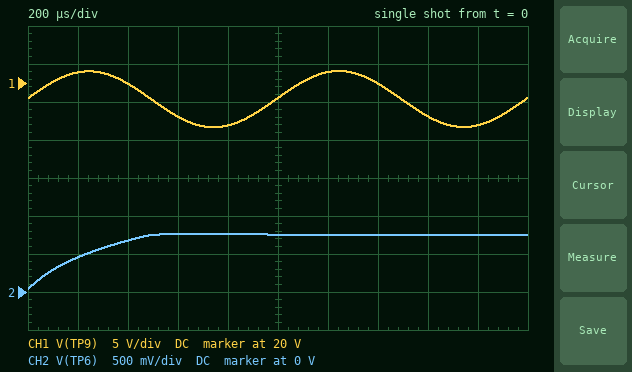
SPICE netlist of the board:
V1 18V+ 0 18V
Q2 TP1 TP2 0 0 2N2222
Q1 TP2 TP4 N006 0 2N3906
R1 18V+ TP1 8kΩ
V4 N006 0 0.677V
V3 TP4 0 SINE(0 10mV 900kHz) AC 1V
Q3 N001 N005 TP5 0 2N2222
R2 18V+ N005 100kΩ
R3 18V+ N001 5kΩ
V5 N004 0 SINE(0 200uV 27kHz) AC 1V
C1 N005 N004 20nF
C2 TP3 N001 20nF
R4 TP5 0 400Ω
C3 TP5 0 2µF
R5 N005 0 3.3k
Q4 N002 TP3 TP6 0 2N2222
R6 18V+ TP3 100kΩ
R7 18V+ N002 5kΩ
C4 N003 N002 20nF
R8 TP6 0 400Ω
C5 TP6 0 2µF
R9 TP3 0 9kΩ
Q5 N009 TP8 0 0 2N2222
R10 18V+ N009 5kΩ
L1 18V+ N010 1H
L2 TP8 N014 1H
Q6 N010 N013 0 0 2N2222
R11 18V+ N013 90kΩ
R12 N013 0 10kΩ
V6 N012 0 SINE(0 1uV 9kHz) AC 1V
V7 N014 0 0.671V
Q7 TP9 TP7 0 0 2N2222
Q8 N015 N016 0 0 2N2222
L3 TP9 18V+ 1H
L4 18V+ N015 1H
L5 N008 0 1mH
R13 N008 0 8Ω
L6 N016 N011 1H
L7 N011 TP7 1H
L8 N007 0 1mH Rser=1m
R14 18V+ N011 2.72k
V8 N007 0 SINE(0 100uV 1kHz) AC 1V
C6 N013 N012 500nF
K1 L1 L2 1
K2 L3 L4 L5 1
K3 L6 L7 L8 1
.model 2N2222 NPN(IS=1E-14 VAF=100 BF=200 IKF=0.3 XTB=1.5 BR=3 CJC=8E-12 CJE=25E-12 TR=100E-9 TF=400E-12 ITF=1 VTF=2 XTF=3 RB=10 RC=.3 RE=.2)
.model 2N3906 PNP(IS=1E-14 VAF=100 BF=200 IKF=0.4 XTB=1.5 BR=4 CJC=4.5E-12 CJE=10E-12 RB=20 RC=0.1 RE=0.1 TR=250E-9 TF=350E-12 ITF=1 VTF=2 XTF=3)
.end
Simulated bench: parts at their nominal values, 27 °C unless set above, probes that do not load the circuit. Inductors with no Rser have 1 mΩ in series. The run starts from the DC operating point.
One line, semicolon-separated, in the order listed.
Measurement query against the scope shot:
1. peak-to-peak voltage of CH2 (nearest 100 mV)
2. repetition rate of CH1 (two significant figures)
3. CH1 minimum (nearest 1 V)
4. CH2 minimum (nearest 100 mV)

700 mV; 1.0 kHz; 14 V; 0 V
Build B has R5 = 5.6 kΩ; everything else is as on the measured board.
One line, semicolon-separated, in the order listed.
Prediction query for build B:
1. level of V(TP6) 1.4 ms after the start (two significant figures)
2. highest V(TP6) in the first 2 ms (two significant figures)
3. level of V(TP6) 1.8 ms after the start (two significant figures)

800 mV; 890 mV; 760 mV
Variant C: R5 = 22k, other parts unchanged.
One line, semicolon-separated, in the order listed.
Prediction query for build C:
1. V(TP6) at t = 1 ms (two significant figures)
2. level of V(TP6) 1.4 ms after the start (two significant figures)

700 mV; 780 mV
